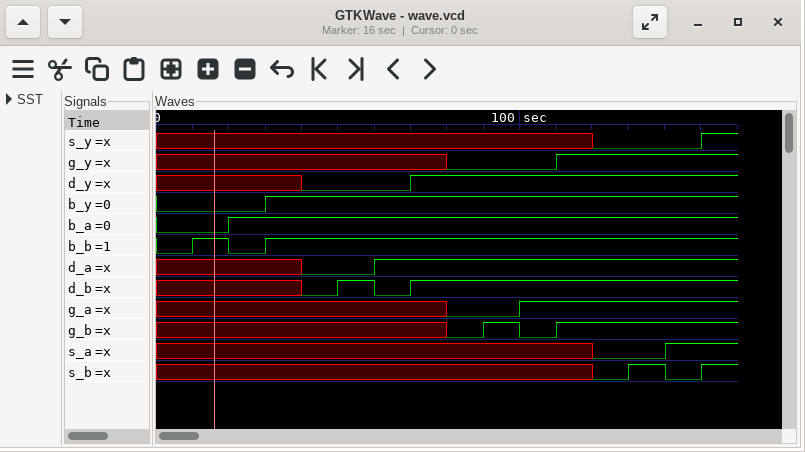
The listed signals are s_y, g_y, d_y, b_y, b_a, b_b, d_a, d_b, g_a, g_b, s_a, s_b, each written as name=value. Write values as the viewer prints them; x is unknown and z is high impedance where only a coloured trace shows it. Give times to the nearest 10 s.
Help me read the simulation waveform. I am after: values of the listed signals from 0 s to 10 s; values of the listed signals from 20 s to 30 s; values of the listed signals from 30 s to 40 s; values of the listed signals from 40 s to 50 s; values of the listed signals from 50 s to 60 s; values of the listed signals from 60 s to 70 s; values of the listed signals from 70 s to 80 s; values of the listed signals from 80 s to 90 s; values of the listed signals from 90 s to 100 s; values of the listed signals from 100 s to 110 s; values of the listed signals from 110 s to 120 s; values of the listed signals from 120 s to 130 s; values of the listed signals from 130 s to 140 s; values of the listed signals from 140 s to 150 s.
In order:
s_y=x, g_y=x, d_y=x, b_y=0, b_a=0, b_b=0, d_a=x, d_b=x, g_a=x, g_b=x, s_a=x, s_b=x
s_y=x, g_y=x, d_y=x, b_y=0, b_a=1, b_b=0, d_a=x, d_b=x, g_a=x, g_b=x, s_a=x, s_b=x
s_y=x, g_y=x, d_y=x, b_y=1, b_a=1, b_b=1, d_a=x, d_b=x, g_a=x, g_b=x, s_a=x, s_b=x
s_y=x, g_y=x, d_y=0, b_y=1, b_a=1, b_b=1, d_a=0, d_b=0, g_a=x, g_b=x, s_a=x, s_b=x
s_y=x, g_y=x, d_y=0, b_y=1, b_a=1, b_b=1, d_a=0, d_b=1, g_a=x, g_b=x, s_a=x, s_b=x
s_y=x, g_y=x, d_y=0, b_y=1, b_a=1, b_b=1, d_a=1, d_b=0, g_a=x, g_b=x, s_a=x, s_b=x
s_y=x, g_y=x, d_y=1, b_y=1, b_a=1, b_b=1, d_a=1, d_b=1, g_a=x, g_b=x, s_a=x, s_b=x
s_y=x, g_y=0, d_y=1, b_y=1, b_a=1, b_b=1, d_a=1, d_b=1, g_a=0, g_b=0, s_a=x, s_b=x
s_y=x, g_y=0, d_y=1, b_y=1, b_a=1, b_b=1, d_a=1, d_b=1, g_a=0, g_b=1, s_a=x, s_b=x
s_y=x, g_y=0, d_y=1, b_y=1, b_a=1, b_b=1, d_a=1, d_b=1, g_a=1, g_b=0, s_a=x, s_b=x
s_y=x, g_y=1, d_y=1, b_y=1, b_a=1, b_b=1, d_a=1, d_b=1, g_a=1, g_b=1, s_a=x, s_b=x
s_y=0, g_y=1, d_y=1, b_y=1, b_a=1, b_b=1, d_a=1, d_b=1, g_a=1, g_b=1, s_a=0, s_b=0
s_y=0, g_y=1, d_y=1, b_y=1, b_a=1, b_b=1, d_a=1, d_b=1, g_a=1, g_b=1, s_a=0, s_b=1
s_y=0, g_y=1, d_y=1, b_y=1, b_a=1, b_b=1, d_a=1, d_b=1, g_a=1, g_b=1, s_a=1, s_b=0
